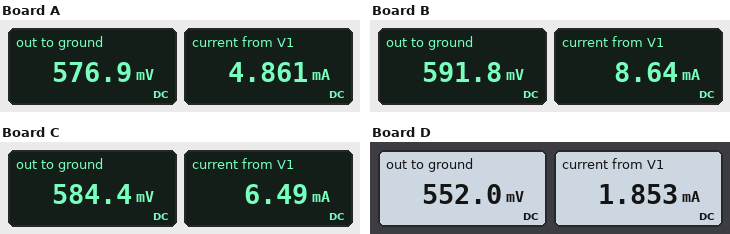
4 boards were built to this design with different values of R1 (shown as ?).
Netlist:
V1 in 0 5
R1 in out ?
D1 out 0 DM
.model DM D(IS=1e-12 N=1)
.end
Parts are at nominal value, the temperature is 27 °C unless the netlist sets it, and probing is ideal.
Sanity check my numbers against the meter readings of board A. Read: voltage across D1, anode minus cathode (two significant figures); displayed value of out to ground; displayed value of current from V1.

580 mV
576.9 mV
4.861 mA
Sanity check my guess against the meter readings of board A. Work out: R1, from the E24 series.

910 Ω
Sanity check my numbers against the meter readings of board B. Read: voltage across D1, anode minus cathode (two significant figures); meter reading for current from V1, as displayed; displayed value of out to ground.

590 mV
8.64 mA
591.8 mV
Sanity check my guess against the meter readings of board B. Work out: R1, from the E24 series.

510 Ω
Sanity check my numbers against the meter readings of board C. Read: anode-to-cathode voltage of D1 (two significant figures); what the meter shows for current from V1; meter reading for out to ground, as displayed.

580 mV
6.49 mA
584.4 mV
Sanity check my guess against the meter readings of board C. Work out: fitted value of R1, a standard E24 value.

680 Ω
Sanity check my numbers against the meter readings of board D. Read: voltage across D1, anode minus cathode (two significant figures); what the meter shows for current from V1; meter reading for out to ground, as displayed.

550 mV
1.853 mA
552.0 mV
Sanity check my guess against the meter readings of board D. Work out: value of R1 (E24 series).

2.4 kΩ
